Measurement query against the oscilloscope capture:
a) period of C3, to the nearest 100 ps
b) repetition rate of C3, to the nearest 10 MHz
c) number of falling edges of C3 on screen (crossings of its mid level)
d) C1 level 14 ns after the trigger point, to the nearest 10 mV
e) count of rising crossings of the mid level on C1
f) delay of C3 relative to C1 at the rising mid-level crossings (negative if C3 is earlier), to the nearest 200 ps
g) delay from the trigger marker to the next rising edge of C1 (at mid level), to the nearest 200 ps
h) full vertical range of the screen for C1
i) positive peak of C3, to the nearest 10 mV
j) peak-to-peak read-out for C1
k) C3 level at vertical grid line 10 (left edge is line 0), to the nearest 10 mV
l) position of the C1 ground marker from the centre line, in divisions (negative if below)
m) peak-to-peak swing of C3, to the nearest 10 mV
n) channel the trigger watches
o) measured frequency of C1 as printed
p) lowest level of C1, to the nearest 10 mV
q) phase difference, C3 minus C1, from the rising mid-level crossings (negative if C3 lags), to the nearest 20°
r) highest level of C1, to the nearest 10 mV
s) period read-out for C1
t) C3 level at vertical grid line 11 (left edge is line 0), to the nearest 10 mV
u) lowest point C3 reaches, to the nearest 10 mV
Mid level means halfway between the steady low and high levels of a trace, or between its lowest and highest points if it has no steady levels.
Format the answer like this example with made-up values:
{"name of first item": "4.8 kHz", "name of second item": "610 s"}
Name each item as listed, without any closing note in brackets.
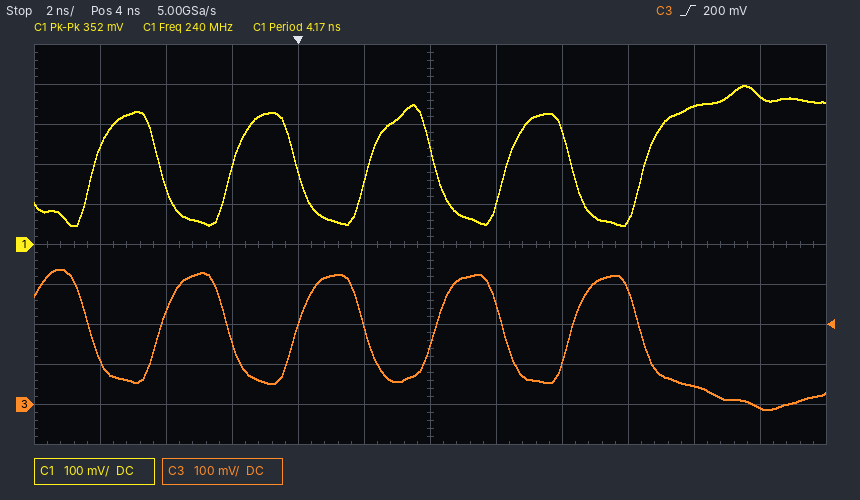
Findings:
{"period of C3, to the nearest 100 ps": "4.2 ns", "repetition rate of C3, to the nearest 10 MHz": "240 MHz", "number of falling edges of C3 on screen": "5", "C1 level 14 ns after the trigger point, to the nearest 10 mV": "370 mV", "count of rising crossings of the mid level on C1": "5", "delay of C3 relative to C1 at the rising mid-level crossings (negative if C3 is earlier), to the nearest 200 ps": "+1.8 ns", "delay from the trigger marker to the next rising edge of C1 (at mid level), to the nearest 200 ps": "2.2 ns", "full vertical range of the screen for C1": "1 V", "positive peak of C3, to the nearest 10 mV": "340 mV", "peak-to-peak read-out for C1": "352 mV", "C3 level at vertical grid line 10 (left edge is line 0), to the nearest 10 mV": "50 mV", "position of the C1 ground marker from the centre line, in divisions": "0.0 div", "peak-to-peak swing of C3, to the nearest 10 mV": "350 mV", "channel the trigger watches": "C3", "measured frequency of C1 as printed": "240 MHz", "lowest level of C1, to the nearest 10 mV": "50 mV", "phase difference, C3 minus C1, from the rising mid-level crossings (negative if C3 lags), to the nearest 20°": "-160°", "highest level of C1, to the nearest 10 mV": "400 mV", "period read-out for C1": "4.17 ns", "C3 level at vertical grid line 11 (left edge is line 0), to the nearest 10 mV": "-10 mV", "lowest point C3 reaches, to the nearest 10 mV": "-10 mV"}
